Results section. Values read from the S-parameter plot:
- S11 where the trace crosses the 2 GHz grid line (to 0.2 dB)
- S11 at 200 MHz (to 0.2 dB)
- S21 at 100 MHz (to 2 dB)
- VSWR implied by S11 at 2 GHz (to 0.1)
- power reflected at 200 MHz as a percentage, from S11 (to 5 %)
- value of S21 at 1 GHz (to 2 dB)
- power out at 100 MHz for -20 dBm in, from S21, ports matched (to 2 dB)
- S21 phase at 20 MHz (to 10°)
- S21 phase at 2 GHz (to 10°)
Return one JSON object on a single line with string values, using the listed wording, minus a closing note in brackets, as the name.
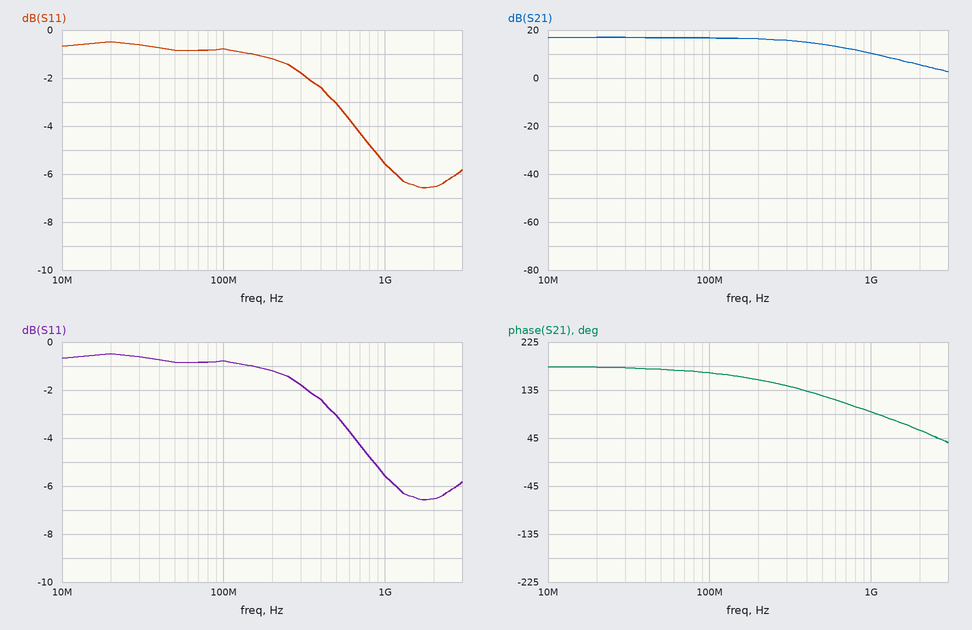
{"S11 where the trace crosses the 2 GHz grid line": "-6.6 dB", "S11 at 200 MHz": "-1.2 dB", "S21 at 100 MHz": "16 dB", "VSWR implied by S11 at 2 GHz": "2.8", "power reflected at 200 MHz as a percentage, from S11": "75 %", "value of S21 at 1 GHz": "10 dB", "power out at 100 MHz for -20 dBm in, from S21, ports matched": "-4 dBm", "S21 phase at 20 MHz": "180°", "S21 phase at 2 GHz": "60°"}
